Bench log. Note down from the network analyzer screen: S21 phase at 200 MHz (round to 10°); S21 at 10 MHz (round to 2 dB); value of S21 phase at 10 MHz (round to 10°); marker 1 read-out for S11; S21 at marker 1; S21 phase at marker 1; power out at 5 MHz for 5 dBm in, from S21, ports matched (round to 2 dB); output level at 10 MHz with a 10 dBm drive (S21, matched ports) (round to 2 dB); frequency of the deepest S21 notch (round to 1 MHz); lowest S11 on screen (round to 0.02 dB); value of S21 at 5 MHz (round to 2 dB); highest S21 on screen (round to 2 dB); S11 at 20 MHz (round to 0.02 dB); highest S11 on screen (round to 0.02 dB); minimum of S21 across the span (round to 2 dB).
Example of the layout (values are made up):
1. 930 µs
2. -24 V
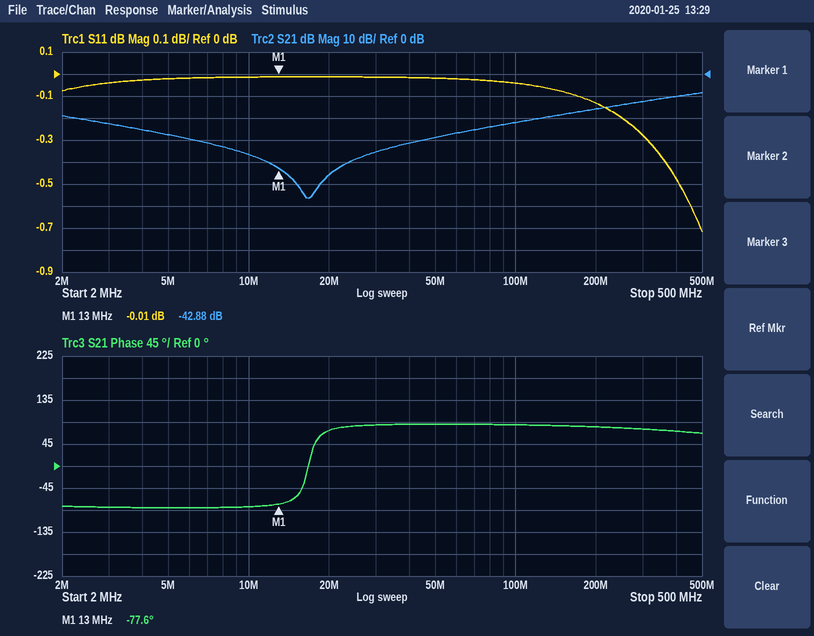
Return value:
1. 80°
2. -36 dB
3. -80°
4. -0.01 dB
5. -42.88 dB
6. -77.6°
7. -22 dBm
8. -26 dBm
9. 17 MHz
10. -0.72 dB
11. -28 dB
12. -8 dB
13. -0.02 dB
14. -0.02 dB
15. -56 dB
